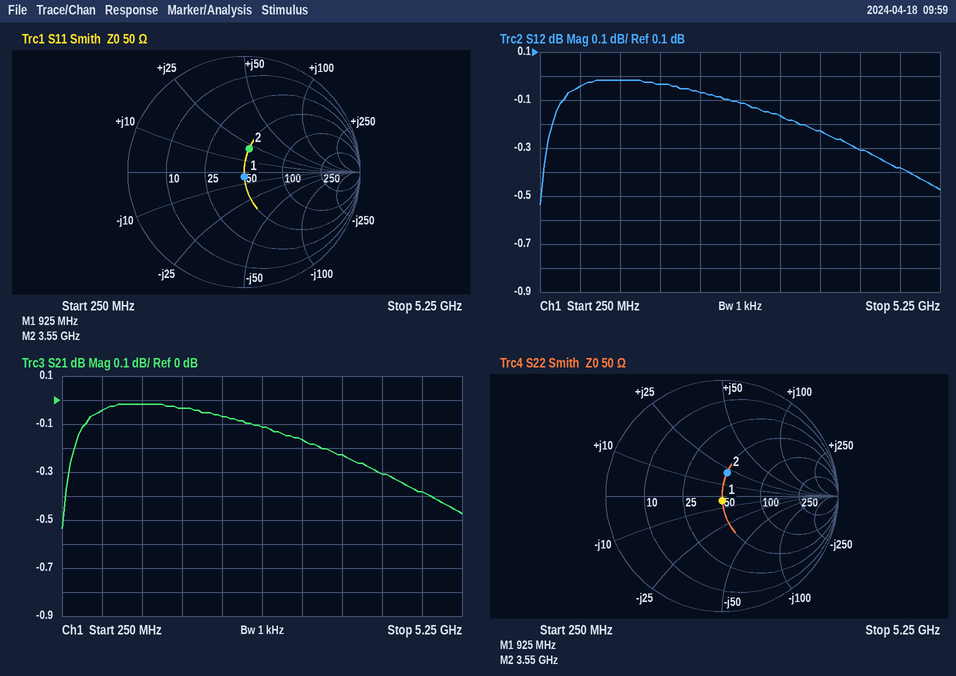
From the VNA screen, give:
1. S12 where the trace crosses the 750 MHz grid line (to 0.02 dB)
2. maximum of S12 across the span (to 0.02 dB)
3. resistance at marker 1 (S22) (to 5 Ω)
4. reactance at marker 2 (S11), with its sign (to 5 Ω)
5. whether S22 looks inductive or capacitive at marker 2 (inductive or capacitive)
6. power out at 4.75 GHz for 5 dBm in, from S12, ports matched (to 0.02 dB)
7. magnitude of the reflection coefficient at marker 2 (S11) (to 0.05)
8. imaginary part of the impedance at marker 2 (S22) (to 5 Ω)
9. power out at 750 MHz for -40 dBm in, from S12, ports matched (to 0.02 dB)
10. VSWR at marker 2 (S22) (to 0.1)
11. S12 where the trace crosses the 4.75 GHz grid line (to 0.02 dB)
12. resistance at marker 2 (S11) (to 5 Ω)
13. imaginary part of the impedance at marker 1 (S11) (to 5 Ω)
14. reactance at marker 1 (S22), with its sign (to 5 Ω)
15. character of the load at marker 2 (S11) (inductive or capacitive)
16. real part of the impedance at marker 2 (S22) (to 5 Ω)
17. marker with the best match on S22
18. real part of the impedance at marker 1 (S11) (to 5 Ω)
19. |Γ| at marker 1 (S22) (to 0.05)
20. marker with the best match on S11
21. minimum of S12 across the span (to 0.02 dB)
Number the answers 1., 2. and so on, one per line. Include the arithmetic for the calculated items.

1. -0.04 dB
2. -0.02 dB
3. 50 Ω
4. +20 Ω
5. inductive
6. 5 dBm + (-0.38 dB) = 4.62 dBm
7. 0.20
8. +20 Ω
9. -40 dBm + (-0.04 dB) = -40.04 dBm
10. 1.5
11. -0.38 dB
12. 50 Ω
13. -5 Ω
14. -5 Ω
15. inductive
16. 50 Ω
17. marker 1
18. 50 Ω
19. 0.05
20. marker 1
21. -0.54 dB
